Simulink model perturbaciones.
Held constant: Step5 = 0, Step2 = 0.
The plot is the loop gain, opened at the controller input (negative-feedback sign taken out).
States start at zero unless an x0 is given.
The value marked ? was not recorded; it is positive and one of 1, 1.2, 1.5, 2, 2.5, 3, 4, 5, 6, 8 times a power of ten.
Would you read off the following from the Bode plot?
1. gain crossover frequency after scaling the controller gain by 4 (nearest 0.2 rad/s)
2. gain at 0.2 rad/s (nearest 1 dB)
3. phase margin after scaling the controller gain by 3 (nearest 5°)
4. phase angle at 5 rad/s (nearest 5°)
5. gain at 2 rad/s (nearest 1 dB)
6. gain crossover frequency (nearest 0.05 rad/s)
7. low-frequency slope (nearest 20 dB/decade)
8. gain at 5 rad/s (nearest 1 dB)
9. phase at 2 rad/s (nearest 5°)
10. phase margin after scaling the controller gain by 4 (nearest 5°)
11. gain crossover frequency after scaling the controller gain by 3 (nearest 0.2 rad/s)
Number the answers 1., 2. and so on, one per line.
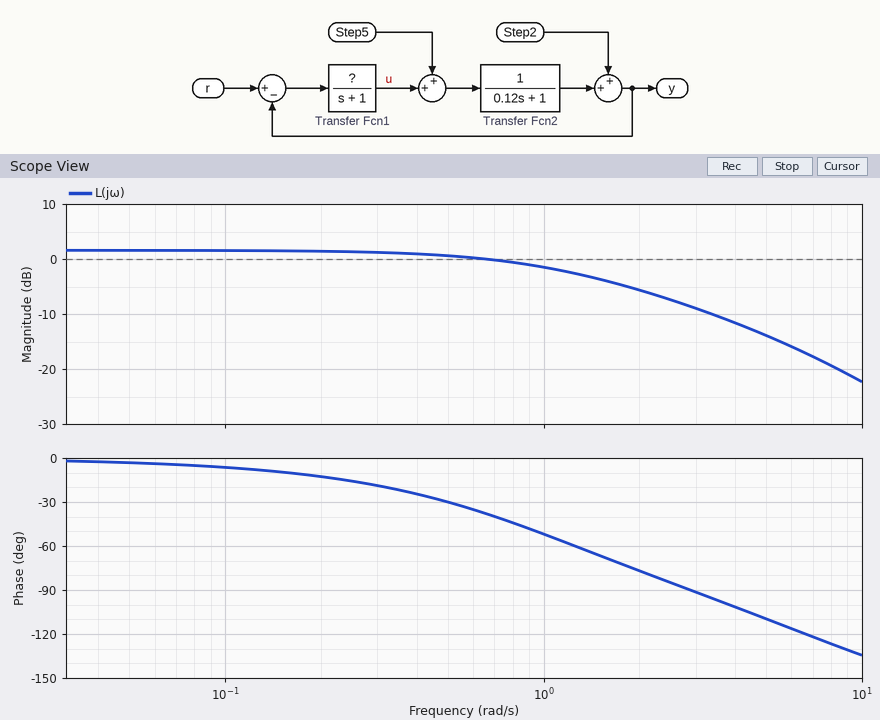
1. 4.2 rad/s
2. 1 dB
3. 85°
4. -110°
5. -6 dB
6. 0.65 rad/s
7. 0 dB/decade
8. -14 dB
9. -75°
10. 75°
11. 3.2 rad/s
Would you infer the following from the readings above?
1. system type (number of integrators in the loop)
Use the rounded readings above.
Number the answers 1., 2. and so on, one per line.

1. 0
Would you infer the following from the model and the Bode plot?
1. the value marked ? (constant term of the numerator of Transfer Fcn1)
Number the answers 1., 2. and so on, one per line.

1. 1.2
